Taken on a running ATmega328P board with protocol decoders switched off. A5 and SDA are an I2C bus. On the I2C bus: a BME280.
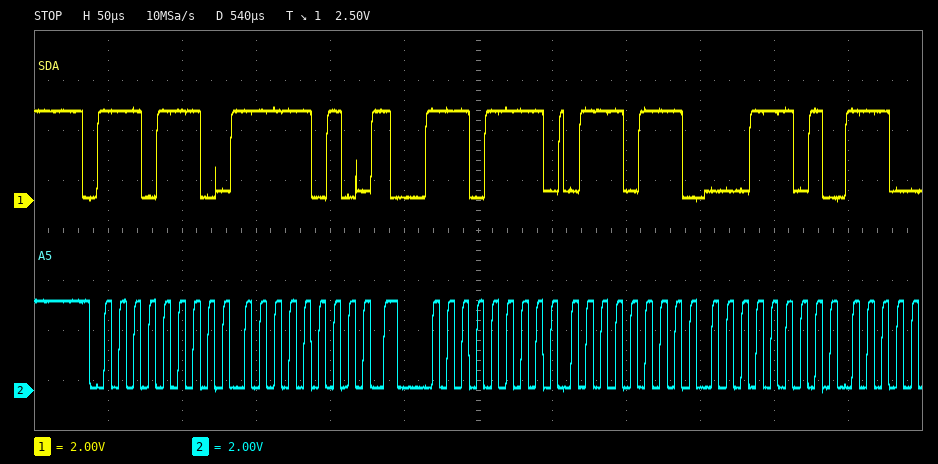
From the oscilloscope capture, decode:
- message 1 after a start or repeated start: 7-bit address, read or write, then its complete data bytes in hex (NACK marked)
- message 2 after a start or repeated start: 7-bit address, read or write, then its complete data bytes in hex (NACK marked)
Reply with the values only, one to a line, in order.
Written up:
0x77 write: FA
0x77 read: 77 1D
